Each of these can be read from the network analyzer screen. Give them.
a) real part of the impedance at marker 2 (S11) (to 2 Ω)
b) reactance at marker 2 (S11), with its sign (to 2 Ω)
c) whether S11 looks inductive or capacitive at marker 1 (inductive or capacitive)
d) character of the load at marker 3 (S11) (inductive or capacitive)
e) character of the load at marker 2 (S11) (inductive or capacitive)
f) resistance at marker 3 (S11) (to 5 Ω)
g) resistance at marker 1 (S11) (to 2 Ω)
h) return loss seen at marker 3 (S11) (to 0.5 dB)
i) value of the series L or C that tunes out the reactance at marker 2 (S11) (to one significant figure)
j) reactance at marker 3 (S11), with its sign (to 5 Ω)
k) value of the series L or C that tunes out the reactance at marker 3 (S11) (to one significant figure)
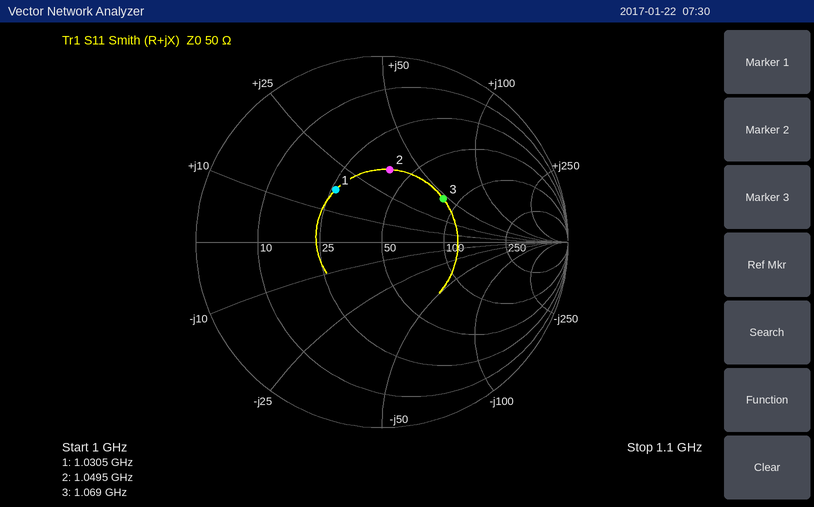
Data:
40 Ω
+36 Ω
inductive
inductive
inductive
85 Ω
26 Ω
8.0 dB
4 pF
+45 Ω
3 pF
